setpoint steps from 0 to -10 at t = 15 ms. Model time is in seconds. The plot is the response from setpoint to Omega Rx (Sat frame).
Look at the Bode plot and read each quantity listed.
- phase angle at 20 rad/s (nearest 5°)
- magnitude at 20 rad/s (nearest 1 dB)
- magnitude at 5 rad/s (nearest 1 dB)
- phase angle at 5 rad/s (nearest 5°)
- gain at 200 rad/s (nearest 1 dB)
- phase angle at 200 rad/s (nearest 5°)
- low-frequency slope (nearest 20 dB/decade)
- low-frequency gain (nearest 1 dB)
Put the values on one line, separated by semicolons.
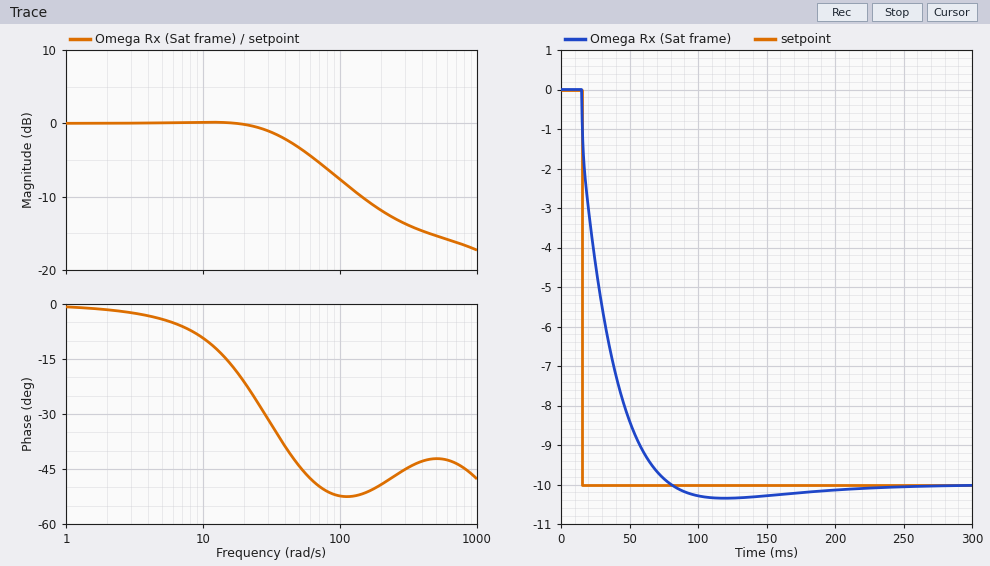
-20°; 0 dB; 0 dB; -5°; -12 dB; -50°; 0 dB/decade; 0 dB
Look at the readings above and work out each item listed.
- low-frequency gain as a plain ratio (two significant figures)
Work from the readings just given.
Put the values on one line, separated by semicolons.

1.0
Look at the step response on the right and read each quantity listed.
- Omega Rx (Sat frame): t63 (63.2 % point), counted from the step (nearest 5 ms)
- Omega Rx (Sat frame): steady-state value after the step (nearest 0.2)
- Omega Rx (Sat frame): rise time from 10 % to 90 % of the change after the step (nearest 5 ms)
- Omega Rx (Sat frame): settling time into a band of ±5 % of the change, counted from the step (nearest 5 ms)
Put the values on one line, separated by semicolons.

20 ms; -10.0; 40 ms; 50 ms
